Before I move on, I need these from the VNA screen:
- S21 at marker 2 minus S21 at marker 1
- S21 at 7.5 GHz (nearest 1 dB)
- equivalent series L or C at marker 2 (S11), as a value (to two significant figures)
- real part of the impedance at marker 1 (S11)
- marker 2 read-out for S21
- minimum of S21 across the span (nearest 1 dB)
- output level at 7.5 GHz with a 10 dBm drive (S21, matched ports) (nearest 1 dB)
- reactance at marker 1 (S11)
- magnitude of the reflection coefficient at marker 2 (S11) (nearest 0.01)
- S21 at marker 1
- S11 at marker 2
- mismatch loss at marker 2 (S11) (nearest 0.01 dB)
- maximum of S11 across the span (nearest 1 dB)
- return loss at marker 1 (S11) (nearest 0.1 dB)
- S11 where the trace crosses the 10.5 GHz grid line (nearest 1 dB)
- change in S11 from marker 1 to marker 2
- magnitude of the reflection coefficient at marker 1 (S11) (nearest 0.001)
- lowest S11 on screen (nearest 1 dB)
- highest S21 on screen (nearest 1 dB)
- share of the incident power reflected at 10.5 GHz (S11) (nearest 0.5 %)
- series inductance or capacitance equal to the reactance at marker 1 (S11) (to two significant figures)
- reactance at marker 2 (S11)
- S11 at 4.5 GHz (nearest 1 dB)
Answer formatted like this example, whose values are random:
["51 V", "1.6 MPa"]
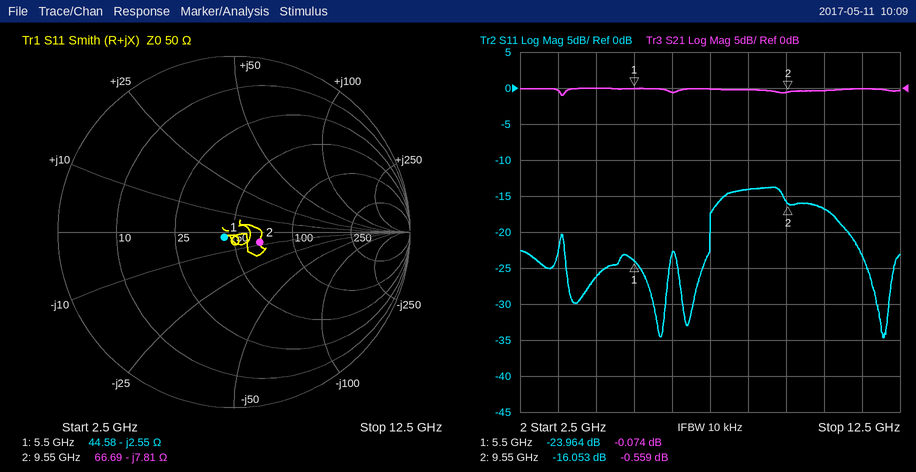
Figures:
["-0.485 dB", "0 dB", "2.1 pF", "44.58 Ω", "-0.559 dB", "-1 dB", "10 dBm", "-2.55 Ω", "0.16", "-0.074 dB", "-16.053 dB", "0.11 dB", "-14 dB", "24.0 dB", "-17 dB", "7.911 dB", "0.063", "-35 dB", "0 dB", "2.0 %", "11 pF", "-7.81 Ω", "-26 dB"]
